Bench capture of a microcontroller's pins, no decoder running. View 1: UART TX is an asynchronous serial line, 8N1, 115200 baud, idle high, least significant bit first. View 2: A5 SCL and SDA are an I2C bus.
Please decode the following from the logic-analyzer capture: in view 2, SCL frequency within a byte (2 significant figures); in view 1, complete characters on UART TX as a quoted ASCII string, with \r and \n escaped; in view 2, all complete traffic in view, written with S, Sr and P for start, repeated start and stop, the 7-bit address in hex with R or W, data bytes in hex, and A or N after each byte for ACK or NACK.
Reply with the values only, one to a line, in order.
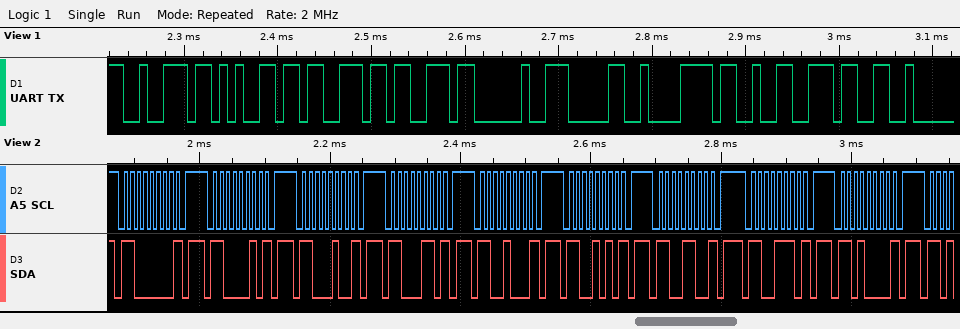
100 kHz
"ress 0x23"
S 60W N P S 61W N P S 62W N P S 63W N P S 64W N P S 65W N P S 66W N P S 67W N P S 68W N P
